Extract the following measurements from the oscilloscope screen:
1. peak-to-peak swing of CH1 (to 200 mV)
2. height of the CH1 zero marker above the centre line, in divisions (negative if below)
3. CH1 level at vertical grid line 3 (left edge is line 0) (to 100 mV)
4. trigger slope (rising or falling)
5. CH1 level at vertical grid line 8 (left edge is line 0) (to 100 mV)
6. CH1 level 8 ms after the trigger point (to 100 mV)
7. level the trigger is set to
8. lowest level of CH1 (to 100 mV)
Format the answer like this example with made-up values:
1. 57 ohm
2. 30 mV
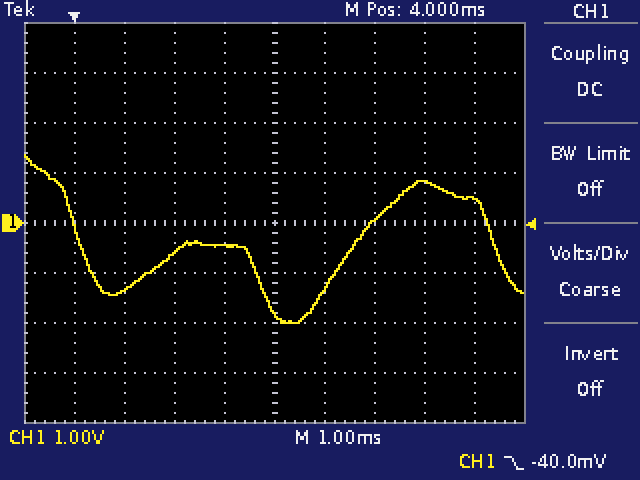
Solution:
1. 3.4 V
2. 0.0 div
3. -600 mV
4. falling
5. 800 mV
6. 500 mV
7. -40.0 mV
8. -2.0 V
